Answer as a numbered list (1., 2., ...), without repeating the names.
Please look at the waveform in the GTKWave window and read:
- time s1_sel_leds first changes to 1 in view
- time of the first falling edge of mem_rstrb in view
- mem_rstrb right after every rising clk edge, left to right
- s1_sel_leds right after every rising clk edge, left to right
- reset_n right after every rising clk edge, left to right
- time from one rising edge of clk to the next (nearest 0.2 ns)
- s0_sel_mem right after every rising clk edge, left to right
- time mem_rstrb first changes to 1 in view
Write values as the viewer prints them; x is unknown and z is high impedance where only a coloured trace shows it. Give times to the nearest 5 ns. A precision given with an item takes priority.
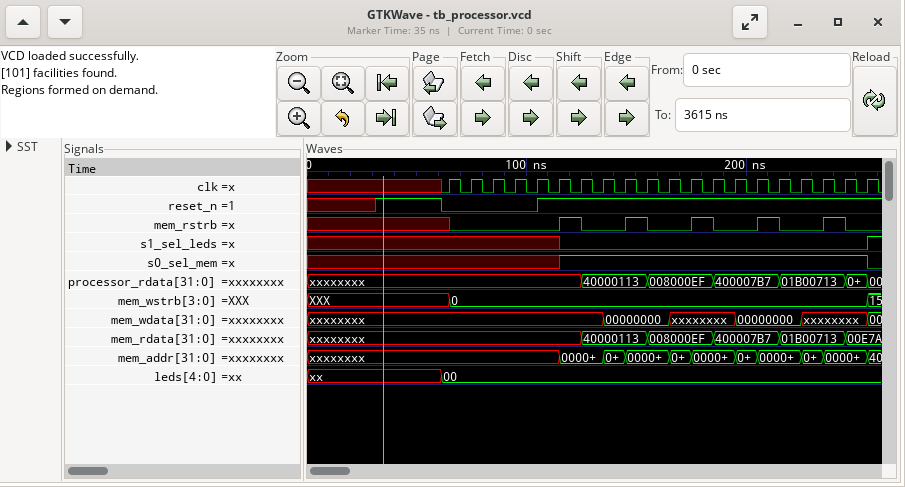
1. 255 ns
2. 125 ns
3. 0 0 0 0 0 1 0 0 1 0 0 1 0 0 1 0 0 1 0 0
4. x x x x x 0 0 0 0 0 0 0 0 0 0 0 0 0 0 1
5. 0 0 0 0 1 1 1 1 1 1 1 1 1 1 1 1 1 1 1 1
6. 10 ns
7. x x x x x 1 1 1 1 1 1 1 1 1 1 1 1 1 1 0
8. 115 ns
